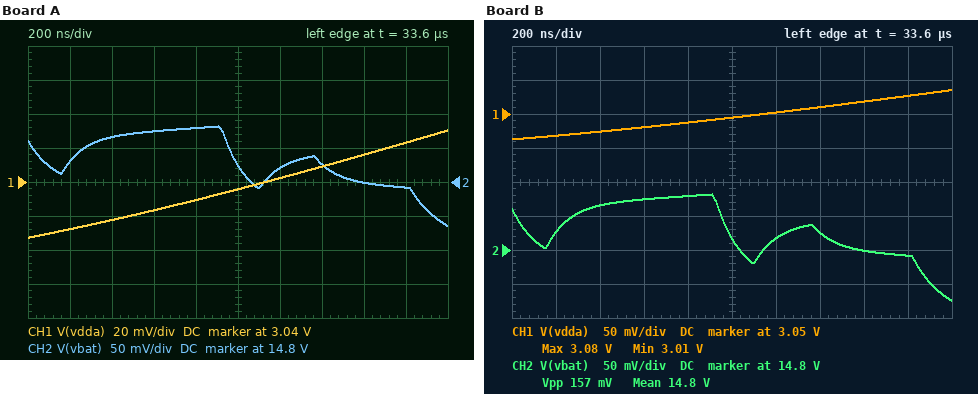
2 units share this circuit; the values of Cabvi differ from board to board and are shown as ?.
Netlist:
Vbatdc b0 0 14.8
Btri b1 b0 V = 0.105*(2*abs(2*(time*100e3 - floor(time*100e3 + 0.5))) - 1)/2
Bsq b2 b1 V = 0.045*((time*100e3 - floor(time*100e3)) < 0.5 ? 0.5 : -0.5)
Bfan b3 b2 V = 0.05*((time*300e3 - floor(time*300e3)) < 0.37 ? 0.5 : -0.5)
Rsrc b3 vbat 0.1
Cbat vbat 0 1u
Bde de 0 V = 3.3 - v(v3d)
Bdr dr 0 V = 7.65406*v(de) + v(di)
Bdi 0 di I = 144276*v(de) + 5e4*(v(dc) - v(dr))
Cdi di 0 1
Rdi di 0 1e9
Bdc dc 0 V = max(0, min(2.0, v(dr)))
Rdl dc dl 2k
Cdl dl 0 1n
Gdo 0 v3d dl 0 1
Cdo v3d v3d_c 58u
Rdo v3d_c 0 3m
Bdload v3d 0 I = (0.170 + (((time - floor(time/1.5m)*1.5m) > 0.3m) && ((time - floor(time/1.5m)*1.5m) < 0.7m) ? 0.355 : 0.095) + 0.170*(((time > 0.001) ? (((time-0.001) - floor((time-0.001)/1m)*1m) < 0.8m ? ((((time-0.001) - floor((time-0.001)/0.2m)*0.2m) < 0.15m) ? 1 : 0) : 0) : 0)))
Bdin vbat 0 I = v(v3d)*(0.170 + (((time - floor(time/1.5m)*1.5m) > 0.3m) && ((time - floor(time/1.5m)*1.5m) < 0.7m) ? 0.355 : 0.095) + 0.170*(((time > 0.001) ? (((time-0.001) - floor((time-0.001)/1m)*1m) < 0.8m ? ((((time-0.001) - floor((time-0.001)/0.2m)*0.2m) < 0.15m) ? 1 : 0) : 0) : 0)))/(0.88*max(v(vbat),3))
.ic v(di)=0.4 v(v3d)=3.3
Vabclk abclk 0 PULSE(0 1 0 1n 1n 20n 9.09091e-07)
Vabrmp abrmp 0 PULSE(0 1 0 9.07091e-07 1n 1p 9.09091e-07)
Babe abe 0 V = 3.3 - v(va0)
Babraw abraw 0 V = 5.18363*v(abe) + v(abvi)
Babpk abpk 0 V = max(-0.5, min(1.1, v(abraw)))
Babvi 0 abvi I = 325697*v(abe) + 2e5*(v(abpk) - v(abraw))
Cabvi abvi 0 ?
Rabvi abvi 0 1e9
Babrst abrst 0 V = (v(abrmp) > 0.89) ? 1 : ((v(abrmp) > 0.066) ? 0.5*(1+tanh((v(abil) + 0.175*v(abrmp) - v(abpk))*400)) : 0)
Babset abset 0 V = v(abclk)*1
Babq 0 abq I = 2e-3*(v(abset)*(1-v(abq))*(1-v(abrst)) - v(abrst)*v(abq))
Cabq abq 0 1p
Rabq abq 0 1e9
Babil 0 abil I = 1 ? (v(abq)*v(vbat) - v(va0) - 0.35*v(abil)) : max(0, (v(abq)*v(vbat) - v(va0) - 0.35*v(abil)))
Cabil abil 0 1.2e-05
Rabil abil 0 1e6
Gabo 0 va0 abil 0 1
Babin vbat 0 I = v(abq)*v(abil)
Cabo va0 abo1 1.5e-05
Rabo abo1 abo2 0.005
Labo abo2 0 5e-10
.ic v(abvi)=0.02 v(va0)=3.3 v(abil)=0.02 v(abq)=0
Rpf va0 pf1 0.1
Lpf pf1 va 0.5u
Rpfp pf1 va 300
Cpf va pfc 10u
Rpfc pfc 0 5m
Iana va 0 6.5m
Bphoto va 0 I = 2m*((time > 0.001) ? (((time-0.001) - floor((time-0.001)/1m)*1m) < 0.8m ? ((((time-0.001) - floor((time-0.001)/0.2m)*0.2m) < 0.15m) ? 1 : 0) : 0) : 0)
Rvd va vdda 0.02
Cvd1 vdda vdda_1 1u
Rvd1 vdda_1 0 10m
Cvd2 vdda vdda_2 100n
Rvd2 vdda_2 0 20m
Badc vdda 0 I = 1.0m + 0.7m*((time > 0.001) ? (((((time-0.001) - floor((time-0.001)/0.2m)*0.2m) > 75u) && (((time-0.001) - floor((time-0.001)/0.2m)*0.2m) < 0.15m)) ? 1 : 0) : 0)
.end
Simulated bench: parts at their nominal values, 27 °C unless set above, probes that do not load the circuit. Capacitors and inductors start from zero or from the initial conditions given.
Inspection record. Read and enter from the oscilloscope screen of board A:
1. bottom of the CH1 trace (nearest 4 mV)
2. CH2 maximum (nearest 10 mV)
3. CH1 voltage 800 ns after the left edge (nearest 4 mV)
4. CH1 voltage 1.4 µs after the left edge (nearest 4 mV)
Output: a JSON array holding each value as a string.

["3.008 V", "14.88 V", "3.028 V", "3.048 V"]
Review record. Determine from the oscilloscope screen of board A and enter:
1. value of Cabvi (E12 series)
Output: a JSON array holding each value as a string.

["820 mF"]
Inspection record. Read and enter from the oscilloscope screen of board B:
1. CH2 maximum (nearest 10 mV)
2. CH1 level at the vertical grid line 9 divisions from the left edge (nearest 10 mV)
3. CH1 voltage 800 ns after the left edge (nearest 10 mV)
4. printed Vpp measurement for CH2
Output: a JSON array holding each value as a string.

["14.88 V", "3.08 V", "3.04 V", "157 mV"]
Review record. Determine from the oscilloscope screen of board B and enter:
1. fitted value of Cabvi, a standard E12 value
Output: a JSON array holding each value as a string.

["560 mF"]
